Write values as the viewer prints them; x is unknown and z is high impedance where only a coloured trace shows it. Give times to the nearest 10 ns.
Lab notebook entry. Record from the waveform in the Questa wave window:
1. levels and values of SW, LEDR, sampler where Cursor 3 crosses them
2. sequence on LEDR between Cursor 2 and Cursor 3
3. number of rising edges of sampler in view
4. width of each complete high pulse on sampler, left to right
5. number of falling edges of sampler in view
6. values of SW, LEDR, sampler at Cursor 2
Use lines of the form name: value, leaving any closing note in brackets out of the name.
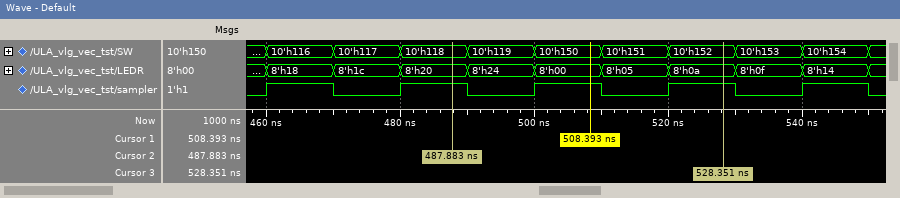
levels and values of SW, LEDR, sampler where Cursor 3 crosses them: SW=10'h152, LEDR=8'h0a, sampler=1
sequence on LEDR between Cursor 2 and Cursor 3: 8'h20, 8'h24, 8'h00, 8'h05, 8'h0a
number of rising edges of sampler in view: 5
width of each complete high pulse on sampler, left to right: 10 ns, 10 ns, 10 ns, 10 ns, 10 ns
number of falling edges of sampler in view: 5
values of SW, LEDR, sampler at Cursor 2: SW=10'h118, LEDR=8'h20, sampler=1
